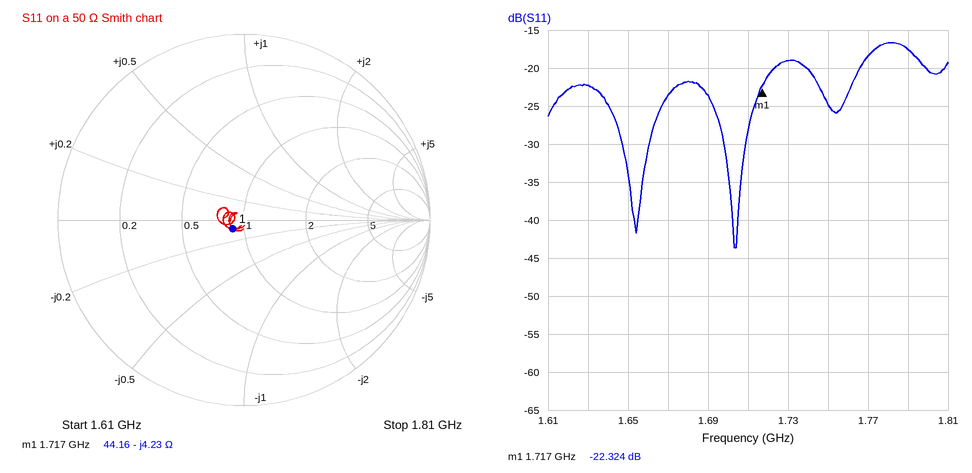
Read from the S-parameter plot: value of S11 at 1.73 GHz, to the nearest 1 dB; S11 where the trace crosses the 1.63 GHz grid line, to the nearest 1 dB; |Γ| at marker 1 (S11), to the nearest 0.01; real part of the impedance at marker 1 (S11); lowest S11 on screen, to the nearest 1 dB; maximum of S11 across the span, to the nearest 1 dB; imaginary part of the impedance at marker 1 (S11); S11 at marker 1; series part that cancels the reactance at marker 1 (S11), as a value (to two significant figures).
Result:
-19 dB
-22 dB
0.08
44.16 Ω
-44 dB
-17 dB
-4.23 Ω
-22.324 dB
390 pH
